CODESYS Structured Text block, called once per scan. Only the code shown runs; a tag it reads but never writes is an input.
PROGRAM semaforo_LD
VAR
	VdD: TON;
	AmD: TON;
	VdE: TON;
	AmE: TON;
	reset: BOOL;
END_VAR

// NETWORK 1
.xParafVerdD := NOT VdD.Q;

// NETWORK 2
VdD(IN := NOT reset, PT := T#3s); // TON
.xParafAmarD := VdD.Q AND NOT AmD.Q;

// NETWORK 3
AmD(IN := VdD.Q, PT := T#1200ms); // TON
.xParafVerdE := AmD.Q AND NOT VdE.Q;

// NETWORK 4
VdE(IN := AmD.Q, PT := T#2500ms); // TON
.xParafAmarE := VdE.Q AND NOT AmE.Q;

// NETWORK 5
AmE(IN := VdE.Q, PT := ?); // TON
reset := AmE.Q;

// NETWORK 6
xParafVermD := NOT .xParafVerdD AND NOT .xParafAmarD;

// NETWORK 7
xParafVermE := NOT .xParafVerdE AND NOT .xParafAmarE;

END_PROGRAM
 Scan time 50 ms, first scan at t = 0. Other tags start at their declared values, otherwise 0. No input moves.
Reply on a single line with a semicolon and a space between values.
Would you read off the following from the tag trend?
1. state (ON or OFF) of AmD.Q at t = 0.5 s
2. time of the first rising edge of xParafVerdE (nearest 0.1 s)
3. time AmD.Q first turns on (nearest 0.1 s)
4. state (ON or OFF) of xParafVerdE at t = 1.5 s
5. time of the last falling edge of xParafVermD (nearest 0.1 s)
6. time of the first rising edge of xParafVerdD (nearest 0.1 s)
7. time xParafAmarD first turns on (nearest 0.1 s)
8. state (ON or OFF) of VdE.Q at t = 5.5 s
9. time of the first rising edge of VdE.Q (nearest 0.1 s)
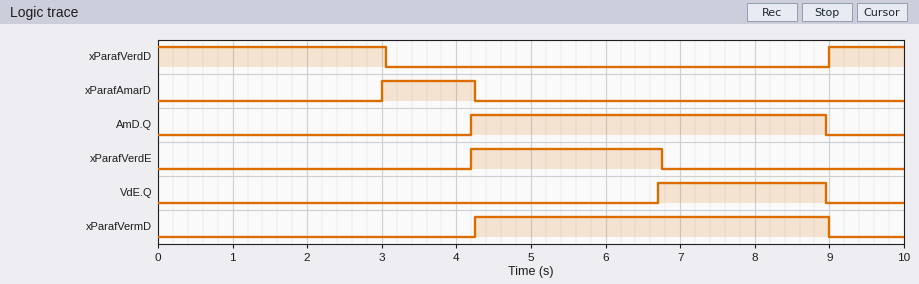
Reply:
OFF; 4.2 s; 4.2 s; OFF; 9.0 s; 9.0 s; 3.0 s; OFF; 6.7 s
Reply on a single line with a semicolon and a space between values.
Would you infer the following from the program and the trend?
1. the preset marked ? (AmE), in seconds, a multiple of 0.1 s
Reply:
2.2 s
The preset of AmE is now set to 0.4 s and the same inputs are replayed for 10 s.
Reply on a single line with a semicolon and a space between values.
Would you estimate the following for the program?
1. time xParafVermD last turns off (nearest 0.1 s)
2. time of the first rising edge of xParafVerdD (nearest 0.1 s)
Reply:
7.2 s; 7.2 s
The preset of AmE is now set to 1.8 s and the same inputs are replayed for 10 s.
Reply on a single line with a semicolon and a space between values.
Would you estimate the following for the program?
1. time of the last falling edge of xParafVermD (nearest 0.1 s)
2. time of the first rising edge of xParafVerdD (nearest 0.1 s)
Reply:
8.6 s; 8.6 s
